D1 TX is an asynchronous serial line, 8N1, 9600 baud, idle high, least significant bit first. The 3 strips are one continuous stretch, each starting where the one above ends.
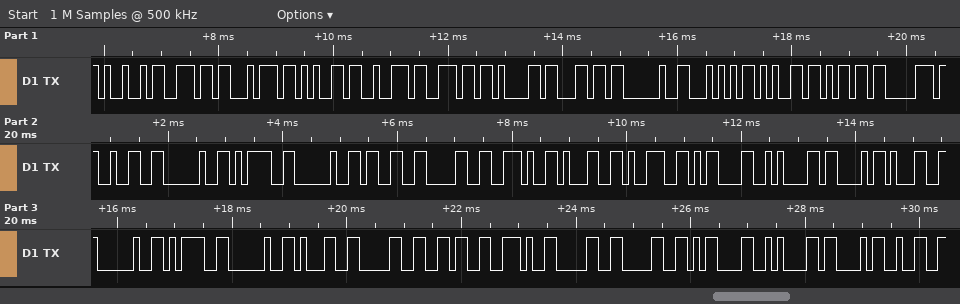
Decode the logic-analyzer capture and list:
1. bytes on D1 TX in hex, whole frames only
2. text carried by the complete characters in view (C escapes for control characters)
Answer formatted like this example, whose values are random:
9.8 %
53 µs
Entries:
49 6E 74 65 72 6E 61 6C 20 54 65 6D 70 32 20 3D 20 33 30 2E 31 39 0D 0A 43 31 20 3D 20 31 30 36 2E 30 30 0D 0A 43 32
"Internal Temp2 = 30.19\r\nC1 = 106.00\r\nC2"
